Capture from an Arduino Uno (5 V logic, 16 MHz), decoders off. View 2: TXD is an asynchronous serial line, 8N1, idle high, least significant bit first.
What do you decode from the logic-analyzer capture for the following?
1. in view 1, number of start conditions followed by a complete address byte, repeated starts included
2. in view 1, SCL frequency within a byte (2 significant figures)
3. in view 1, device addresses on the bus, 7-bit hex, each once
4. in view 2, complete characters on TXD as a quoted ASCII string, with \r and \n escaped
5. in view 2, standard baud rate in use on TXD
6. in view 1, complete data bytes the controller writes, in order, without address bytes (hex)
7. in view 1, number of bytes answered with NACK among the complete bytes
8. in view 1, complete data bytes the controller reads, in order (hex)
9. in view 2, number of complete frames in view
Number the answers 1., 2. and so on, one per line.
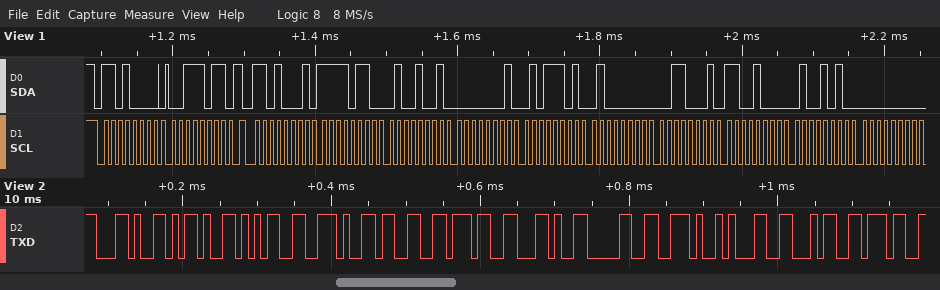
1. 2
2. 100 kHz
3. 0x68
4. ",-5.37,0.147"
5. 115200 baud
6. 3B
7. 0
8. F6 49 01 5D 40 31 C8 4A 00
9. 12
